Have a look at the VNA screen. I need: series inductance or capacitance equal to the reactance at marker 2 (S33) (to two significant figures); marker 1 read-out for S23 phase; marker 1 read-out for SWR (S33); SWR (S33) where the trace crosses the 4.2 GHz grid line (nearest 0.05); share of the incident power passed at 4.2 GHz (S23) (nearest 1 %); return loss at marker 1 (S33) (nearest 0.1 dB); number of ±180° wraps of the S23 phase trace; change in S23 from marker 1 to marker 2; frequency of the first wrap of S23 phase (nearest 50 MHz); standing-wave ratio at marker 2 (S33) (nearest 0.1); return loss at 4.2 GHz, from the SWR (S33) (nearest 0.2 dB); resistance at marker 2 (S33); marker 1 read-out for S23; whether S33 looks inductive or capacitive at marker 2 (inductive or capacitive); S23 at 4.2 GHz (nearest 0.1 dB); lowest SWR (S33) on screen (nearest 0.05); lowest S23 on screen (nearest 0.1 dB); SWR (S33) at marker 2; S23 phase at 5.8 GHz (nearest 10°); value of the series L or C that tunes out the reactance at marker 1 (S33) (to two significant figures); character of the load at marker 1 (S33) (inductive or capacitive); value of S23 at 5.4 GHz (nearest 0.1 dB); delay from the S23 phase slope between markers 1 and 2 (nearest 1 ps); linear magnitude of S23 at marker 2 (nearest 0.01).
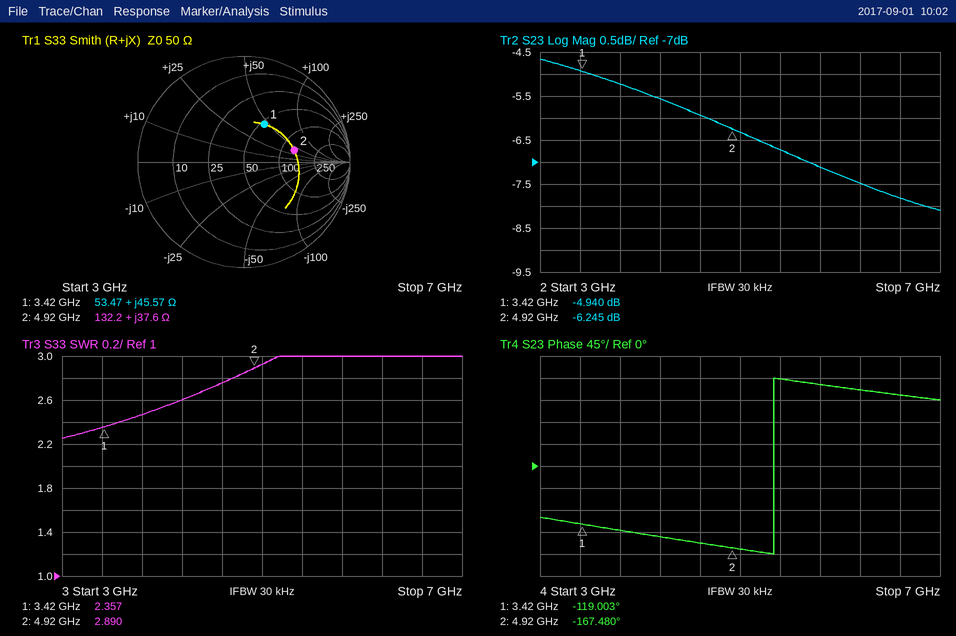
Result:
1.2 nH
-119.003°
2.357
2.60
28 %
7.9 dB
1
-1.305 dB
5.35 GHz
2.9
7.0 dB
132.2 Ω
-4.940 dB
inductive
-5.6 dB
2.25
-8.1 dB
2.890
170°
1.0 pF
inductive
-6.7 dB
90 ps
0.49
